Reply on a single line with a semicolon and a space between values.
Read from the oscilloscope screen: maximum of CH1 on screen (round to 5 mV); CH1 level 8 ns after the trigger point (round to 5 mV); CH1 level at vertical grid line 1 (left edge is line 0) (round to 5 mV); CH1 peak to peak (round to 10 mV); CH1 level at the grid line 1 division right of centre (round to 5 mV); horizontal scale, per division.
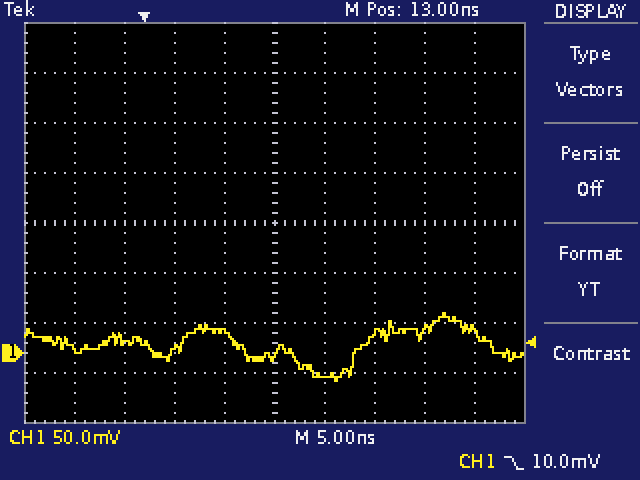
40 mV; 20 mV; 5 mV; 70 mV; -25 mV; 5 ns
